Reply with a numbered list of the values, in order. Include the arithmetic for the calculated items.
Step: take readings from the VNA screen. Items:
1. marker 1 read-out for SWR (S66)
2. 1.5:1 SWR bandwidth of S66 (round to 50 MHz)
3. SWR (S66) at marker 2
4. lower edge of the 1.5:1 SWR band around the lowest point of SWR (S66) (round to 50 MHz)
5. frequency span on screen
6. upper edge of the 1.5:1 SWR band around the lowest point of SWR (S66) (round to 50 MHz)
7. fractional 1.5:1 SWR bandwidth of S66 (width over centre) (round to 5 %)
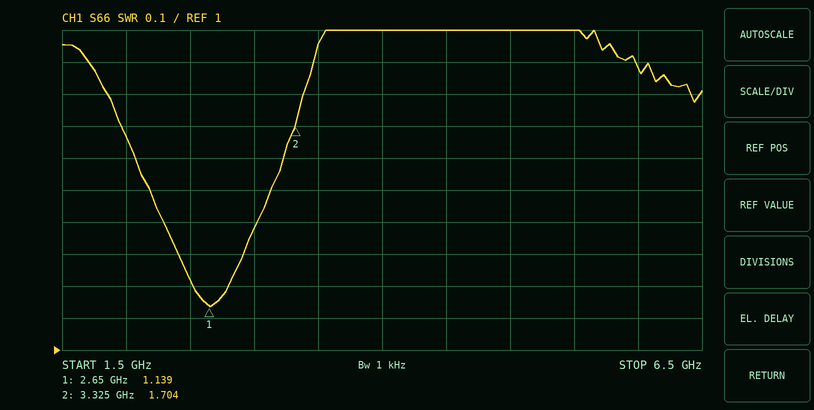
1. 1.139
2. 3.15 GHz − 2.20 GHz = 950 MHz
3. 1.704
4. 2.20 GHz
5. 5 GHz
6. 3.15 GHz
7. 950 MHz / 2.675 GHz ≈ 35 %
